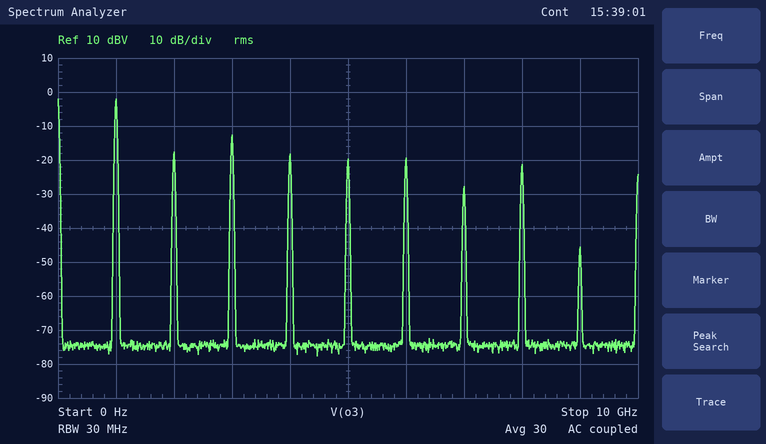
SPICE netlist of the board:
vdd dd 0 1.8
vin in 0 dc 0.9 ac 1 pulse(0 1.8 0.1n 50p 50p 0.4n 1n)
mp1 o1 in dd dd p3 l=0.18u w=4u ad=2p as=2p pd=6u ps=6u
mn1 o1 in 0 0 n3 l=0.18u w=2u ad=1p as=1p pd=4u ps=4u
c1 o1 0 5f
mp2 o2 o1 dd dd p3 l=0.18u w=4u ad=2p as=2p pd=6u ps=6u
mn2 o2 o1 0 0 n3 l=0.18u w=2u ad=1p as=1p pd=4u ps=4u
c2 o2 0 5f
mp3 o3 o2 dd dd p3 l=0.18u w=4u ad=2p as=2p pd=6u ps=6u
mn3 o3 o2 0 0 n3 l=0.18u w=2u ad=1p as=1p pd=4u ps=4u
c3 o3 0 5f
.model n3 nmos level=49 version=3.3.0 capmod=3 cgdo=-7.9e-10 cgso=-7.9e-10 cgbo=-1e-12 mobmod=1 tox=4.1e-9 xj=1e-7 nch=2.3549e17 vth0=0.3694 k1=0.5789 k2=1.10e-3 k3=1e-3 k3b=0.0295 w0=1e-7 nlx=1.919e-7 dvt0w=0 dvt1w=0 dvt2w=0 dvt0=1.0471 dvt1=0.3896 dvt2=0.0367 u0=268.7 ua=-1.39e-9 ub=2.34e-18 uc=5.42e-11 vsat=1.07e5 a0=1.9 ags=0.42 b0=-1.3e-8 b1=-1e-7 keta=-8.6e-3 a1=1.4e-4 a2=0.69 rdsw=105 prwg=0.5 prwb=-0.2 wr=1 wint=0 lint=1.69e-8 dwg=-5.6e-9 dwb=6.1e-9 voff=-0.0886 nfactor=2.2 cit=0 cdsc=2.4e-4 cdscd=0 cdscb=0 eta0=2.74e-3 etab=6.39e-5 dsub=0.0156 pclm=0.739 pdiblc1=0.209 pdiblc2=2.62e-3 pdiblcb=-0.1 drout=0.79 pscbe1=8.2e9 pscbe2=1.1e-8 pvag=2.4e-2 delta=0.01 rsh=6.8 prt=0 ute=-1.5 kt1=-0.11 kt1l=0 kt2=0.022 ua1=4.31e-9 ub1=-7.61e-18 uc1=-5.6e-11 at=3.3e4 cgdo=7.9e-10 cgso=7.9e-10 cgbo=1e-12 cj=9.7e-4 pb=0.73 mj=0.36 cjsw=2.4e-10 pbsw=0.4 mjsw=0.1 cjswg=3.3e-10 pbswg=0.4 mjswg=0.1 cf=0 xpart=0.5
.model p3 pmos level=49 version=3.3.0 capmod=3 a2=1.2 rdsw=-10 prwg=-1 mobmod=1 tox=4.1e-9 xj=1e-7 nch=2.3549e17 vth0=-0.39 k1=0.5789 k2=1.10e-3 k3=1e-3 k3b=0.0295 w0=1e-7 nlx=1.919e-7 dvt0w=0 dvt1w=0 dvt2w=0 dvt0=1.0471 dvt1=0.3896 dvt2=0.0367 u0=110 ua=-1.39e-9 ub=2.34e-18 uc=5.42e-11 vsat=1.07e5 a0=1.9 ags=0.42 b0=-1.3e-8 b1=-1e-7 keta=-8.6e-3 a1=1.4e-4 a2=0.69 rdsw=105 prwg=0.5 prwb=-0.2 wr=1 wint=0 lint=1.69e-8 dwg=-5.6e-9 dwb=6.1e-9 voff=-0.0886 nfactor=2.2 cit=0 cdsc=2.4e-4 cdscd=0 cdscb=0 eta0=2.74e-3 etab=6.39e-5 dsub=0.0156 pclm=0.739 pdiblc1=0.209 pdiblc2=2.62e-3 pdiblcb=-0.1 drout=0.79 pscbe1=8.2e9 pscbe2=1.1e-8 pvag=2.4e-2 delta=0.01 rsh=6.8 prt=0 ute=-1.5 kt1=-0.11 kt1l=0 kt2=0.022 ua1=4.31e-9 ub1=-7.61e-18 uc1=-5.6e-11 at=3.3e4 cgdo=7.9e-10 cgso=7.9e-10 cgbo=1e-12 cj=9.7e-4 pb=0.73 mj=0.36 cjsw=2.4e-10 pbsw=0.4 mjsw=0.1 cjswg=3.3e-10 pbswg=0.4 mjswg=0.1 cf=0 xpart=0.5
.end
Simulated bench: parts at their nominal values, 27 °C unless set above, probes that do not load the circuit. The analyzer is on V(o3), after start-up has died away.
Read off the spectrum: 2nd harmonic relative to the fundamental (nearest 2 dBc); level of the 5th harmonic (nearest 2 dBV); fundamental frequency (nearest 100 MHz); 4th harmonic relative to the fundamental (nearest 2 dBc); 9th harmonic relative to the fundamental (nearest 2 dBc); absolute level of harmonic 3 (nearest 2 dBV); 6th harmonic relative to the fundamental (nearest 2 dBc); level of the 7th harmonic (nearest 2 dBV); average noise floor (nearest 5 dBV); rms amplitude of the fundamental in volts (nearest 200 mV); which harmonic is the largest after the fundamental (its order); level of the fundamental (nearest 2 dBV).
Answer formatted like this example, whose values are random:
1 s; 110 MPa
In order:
-16 dBc; -20 dBV; 1.0 GHz; -16 dBc; -44 dBc; -12 dBV; -18 dBc; -28 dBV; -75 dBV; 800 mV; 3; -2 dBV
